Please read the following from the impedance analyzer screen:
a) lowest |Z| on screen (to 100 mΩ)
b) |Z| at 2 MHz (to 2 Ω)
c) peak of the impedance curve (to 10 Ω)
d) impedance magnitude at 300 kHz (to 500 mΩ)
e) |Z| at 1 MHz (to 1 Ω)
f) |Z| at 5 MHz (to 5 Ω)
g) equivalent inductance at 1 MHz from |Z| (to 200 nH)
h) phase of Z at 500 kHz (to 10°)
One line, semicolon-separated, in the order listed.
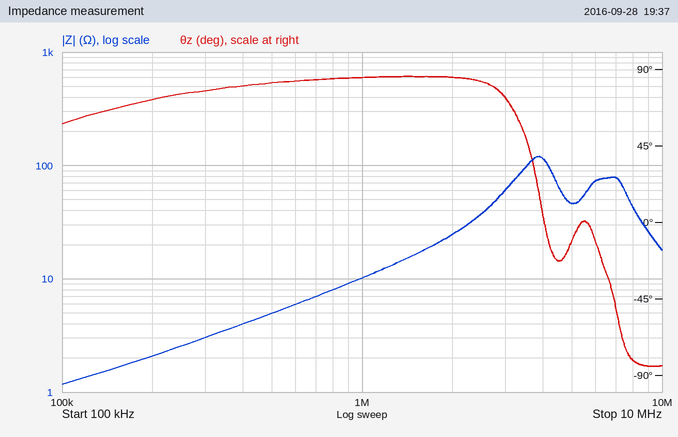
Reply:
1.2 Ω; 24 Ω; 120 Ω; 3.0 Ω; 10 Ω; 45 Ω; 1.6 µH; 80°
